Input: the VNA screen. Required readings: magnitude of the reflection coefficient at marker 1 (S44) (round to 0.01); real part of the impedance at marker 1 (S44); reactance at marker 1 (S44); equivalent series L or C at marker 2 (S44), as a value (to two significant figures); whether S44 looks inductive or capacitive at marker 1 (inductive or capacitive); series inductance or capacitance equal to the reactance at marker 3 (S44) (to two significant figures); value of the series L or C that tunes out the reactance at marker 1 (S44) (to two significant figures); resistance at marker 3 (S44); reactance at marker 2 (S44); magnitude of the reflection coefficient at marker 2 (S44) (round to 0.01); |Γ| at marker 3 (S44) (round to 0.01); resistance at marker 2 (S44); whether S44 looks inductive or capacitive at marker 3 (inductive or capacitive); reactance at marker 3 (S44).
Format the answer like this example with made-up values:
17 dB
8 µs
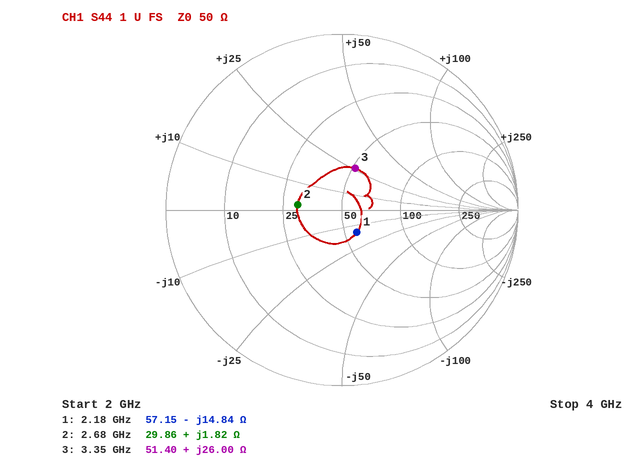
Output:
0.15
57.15 Ω
-14.84 Ω
110 pH
capacitive
1.2 nH
1.1 nH
51.40 Ω
+1.82 Ω
0.25
0.25
29.86 Ω
inductive
+26.00 Ω
